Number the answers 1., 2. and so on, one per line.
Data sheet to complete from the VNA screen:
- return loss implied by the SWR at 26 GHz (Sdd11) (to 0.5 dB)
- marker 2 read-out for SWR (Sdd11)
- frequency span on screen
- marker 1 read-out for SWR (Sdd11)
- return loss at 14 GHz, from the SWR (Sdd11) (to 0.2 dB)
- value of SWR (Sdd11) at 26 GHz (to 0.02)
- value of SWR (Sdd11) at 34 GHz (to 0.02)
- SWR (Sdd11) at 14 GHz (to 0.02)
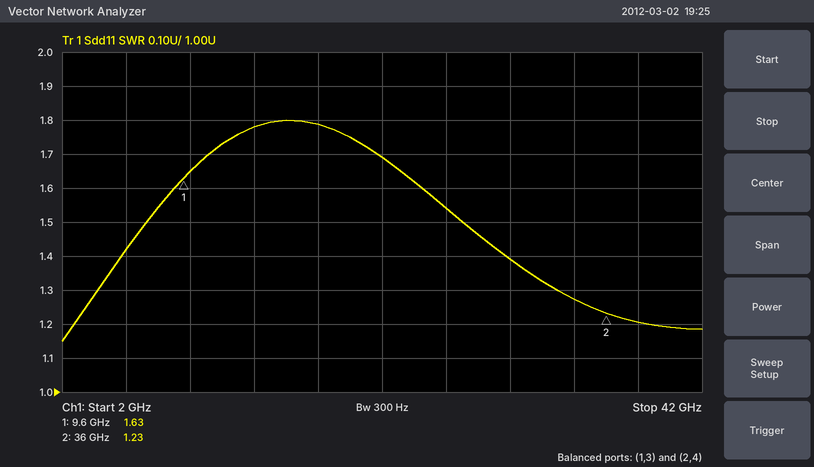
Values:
1. 13.5 dB
2. 1.23
3. 40 GHz
4. 1.63
5. 11.0 dB
6. 1.54
7. 1.28
8. 1.78
